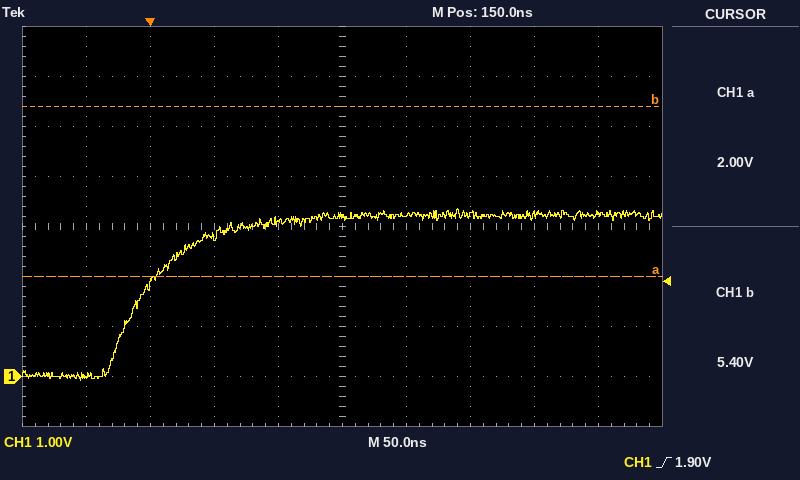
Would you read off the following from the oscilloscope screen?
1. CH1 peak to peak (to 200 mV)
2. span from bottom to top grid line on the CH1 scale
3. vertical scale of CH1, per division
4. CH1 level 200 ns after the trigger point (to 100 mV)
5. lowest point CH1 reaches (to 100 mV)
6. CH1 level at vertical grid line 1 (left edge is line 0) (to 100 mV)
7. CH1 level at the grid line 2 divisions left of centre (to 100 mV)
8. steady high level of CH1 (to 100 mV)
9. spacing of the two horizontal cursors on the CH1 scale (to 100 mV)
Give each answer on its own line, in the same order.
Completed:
3.4 V
8 V
1 V
3.2 V
-100 mV
0.0 V
2.8 V
3.2 V
3.4 V
